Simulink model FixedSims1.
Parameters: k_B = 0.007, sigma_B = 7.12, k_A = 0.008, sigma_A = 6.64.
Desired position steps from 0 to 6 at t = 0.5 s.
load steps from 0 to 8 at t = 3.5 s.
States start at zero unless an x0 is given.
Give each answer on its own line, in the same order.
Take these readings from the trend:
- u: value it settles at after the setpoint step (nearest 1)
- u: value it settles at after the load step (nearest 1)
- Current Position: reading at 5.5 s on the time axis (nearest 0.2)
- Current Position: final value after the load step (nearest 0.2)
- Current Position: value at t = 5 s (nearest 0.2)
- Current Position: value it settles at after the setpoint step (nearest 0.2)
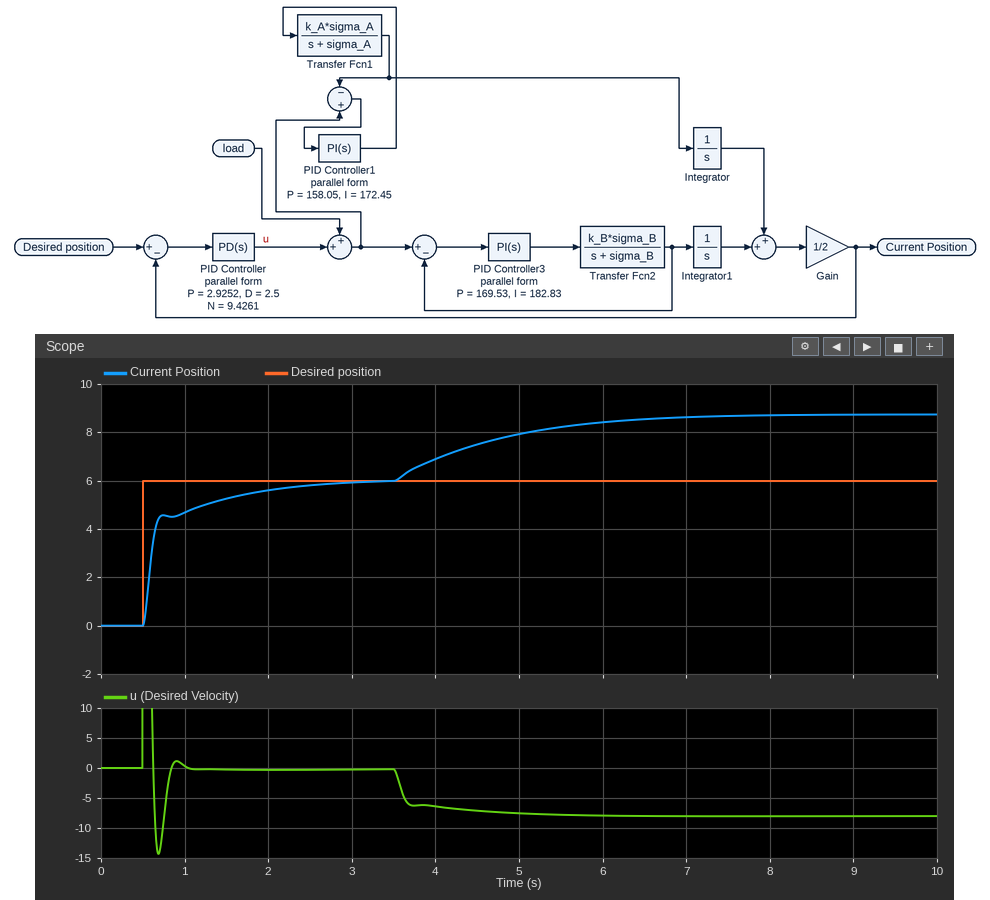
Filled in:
0
-8
8.2
8.8
8.0
6.0
